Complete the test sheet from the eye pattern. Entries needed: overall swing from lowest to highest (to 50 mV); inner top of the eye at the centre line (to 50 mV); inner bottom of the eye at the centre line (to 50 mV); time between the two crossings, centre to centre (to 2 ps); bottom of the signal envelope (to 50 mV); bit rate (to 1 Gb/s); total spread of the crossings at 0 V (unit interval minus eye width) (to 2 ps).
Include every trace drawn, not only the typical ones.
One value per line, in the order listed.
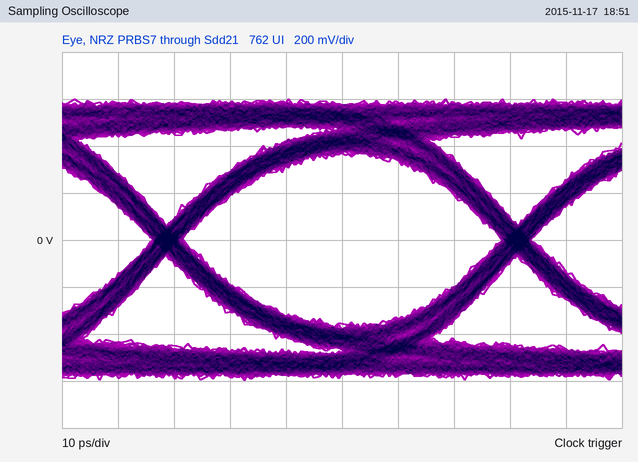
1.20 V
350 mV
-350 mV
62 ps
-600 mV
16 Gb/s
6 ps
